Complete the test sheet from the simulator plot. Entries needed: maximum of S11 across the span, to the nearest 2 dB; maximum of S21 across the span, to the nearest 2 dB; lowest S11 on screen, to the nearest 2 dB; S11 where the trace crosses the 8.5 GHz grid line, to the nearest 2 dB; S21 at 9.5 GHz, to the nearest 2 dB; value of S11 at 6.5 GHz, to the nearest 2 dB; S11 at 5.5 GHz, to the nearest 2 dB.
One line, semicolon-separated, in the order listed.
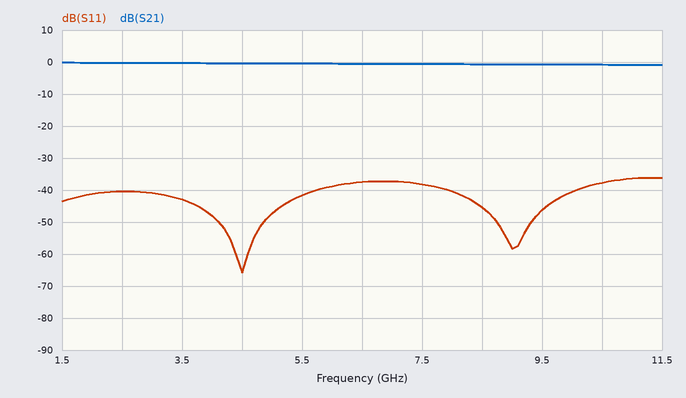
-36 dB; 0 dB; -66 dB; -46 dB; 0 dB; -38 dB; -42 dB
